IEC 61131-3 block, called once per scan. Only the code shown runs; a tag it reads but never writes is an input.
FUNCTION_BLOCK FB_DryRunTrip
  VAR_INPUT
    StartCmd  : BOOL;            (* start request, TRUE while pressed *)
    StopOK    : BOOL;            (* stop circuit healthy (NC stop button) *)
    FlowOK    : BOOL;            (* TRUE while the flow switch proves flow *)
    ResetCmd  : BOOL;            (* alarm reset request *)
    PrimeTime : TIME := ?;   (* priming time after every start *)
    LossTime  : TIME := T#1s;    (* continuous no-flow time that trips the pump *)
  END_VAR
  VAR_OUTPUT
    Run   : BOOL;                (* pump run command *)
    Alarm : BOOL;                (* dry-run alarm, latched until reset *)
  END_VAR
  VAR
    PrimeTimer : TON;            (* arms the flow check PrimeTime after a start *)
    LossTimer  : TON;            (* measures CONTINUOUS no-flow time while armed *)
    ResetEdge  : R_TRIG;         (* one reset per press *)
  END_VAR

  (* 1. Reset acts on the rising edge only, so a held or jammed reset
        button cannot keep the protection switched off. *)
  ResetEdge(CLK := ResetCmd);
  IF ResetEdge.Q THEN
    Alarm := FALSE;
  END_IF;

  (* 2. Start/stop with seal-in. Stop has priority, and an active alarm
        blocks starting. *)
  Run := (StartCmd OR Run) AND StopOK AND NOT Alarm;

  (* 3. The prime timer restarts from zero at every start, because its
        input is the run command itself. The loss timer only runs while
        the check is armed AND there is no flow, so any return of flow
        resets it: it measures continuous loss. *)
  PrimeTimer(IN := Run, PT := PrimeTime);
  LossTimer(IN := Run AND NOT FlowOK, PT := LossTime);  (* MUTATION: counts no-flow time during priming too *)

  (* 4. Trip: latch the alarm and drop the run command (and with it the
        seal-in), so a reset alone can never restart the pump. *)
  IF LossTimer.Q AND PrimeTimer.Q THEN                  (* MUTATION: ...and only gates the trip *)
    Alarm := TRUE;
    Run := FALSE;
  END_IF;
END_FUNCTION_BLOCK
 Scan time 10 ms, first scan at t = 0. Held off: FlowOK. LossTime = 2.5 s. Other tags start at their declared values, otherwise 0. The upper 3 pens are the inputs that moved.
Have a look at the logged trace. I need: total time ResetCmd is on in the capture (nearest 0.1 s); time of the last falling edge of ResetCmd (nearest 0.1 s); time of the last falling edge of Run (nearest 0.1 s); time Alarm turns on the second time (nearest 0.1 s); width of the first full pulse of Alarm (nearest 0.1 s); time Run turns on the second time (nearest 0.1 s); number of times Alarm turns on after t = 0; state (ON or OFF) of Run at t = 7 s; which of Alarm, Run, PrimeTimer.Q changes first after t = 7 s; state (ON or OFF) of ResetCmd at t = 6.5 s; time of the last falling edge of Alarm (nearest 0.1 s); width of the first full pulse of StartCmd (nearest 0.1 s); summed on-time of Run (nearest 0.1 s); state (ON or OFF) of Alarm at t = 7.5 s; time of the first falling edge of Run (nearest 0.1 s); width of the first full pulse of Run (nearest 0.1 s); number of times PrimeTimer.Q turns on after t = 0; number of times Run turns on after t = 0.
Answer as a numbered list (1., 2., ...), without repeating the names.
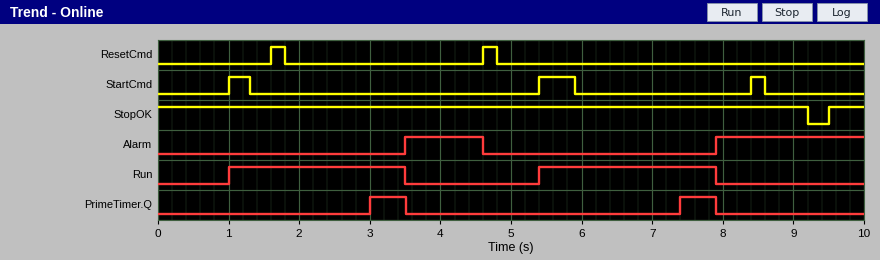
1. 0.4 s
2. 4.8 s
3. 7.9 s
4. 7.9 s
5. 1.1 s
6. 5.4 s
7. 2
8. ON
9. PrimeTimer.Q
10. OFF
11. 4.6 s
12. 0.3 s
13. 5.0 s
14. OFF
15. 3.5 s
16. 2.5 s
17. 2
18. 2
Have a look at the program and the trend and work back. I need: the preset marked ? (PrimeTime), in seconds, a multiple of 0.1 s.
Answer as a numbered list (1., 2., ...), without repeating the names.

1. 2.0 s
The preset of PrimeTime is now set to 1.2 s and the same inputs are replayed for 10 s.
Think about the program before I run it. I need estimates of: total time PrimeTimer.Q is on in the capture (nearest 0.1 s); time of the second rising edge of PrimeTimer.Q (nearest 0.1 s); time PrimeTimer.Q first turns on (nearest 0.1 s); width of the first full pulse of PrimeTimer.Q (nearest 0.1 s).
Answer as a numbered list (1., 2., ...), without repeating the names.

1. 2.6 s
2. 6.6 s
3. 2.2 s
4. 1.3 s
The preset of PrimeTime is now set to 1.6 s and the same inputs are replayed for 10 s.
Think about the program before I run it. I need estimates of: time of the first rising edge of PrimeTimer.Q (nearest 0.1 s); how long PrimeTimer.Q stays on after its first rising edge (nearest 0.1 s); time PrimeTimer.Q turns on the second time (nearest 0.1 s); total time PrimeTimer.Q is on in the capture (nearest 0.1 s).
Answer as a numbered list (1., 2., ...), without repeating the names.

1. 2.6 s
2. 0.9 s
3. 7.0 s
4. 1.8 s
